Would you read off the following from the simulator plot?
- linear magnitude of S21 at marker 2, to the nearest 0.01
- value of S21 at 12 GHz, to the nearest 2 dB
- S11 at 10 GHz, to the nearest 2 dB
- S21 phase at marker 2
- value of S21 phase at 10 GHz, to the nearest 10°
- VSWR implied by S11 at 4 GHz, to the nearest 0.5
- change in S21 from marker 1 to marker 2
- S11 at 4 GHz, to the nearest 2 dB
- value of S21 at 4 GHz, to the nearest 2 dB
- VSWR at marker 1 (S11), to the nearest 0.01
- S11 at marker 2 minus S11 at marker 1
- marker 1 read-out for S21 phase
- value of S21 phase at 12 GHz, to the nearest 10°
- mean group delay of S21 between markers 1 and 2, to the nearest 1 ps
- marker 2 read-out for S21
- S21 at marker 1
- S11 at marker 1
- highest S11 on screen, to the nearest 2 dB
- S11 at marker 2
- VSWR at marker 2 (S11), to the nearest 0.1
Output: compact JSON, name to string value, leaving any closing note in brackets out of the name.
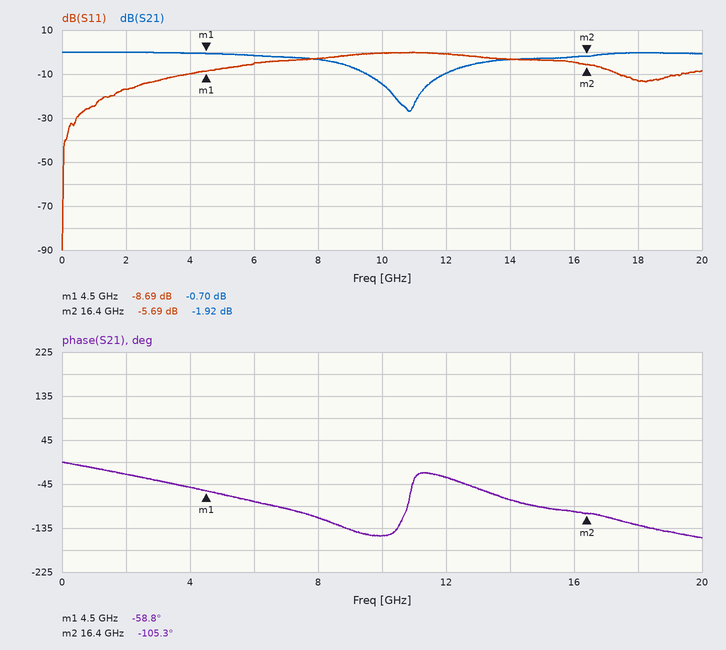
{"linear magnitude of S21 at marker 2, to the nearest 0.01": "0.80", "value of S21 at 12 GHz, to the nearest 2 dB": "-10 dB", "S11 at 10 GHz, to the nearest 2 dB": "0 dB", "S21 phase at marker 2": "-105.3°", "value of S21 phase at 10 GHz, to the nearest 10°": "-150°", "VSWR implied by S11 at 4 GHz, to the nearest 0.5": "2.0", "change in S21 from marker 1 to marker 2": "-1.22 dB", "S11 at 4 GHz, to the nearest 2 dB": "-10 dB", "value of S21 at 4 GHz, to the nearest 2 dB": "0 dB", "VSWR at marker 1 (S11), to the nearest 0.01": "2.16", "S11 at marker 2 minus S11 at marker 1": "3.00 dB", "marker 1 read-out for S21 phase": "-58.8°", "value of S21 phase at 12 GHz, to the nearest 10°": "-30°", "mean group delay of S21 between markers 1 and 2, to the nearest 1 ps": "11 ps", "marker 2 read-out for S21": "-1.92 dB", "S21 at marker 1": "-0.70 dB", "S11 at marker 1": "-8.69 dB", "highest S11 on screen, to the nearest 2 dB": "0 dB", "S11 at marker 2": "-5.69 dB", "VSWR at marker 2 (S11), to the nearest 0.1": "3.2"}
